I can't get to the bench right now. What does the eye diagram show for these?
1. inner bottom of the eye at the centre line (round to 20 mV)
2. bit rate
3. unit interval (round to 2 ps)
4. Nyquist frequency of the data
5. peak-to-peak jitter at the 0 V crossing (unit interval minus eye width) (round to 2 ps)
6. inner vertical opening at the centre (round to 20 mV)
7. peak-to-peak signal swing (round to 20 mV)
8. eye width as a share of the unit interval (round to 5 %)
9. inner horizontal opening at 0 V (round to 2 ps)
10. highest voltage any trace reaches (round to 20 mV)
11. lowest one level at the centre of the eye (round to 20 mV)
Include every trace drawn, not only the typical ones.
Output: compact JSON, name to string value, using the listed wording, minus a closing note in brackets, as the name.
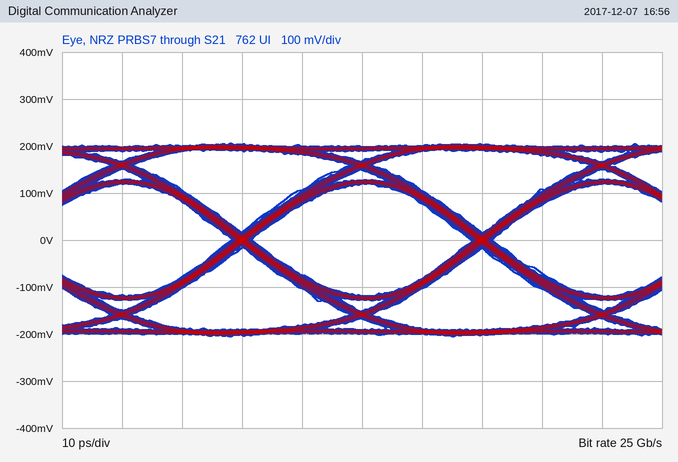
{"inner bottom of the eye at the centre line": "-120 mV", "bit rate": "25 Gb/s", "unit interval": "40 ps", "Nyquist frequency of the data": "12.5 GHz", "peak-to-peak jitter at the 0 V crossing (unit interval minus eye width)": "4 ps", "inner vertical opening at the centre": "240 mV", "peak-to-peak signal swing": "420 mV", "eye width as a share of the unit interval": "90 %", "inner horizontal opening at 0 V": "36 ps", "highest voltage any trace reaches": "200 mV", "lowest one level at the centre of the eye": "120 mV"}
